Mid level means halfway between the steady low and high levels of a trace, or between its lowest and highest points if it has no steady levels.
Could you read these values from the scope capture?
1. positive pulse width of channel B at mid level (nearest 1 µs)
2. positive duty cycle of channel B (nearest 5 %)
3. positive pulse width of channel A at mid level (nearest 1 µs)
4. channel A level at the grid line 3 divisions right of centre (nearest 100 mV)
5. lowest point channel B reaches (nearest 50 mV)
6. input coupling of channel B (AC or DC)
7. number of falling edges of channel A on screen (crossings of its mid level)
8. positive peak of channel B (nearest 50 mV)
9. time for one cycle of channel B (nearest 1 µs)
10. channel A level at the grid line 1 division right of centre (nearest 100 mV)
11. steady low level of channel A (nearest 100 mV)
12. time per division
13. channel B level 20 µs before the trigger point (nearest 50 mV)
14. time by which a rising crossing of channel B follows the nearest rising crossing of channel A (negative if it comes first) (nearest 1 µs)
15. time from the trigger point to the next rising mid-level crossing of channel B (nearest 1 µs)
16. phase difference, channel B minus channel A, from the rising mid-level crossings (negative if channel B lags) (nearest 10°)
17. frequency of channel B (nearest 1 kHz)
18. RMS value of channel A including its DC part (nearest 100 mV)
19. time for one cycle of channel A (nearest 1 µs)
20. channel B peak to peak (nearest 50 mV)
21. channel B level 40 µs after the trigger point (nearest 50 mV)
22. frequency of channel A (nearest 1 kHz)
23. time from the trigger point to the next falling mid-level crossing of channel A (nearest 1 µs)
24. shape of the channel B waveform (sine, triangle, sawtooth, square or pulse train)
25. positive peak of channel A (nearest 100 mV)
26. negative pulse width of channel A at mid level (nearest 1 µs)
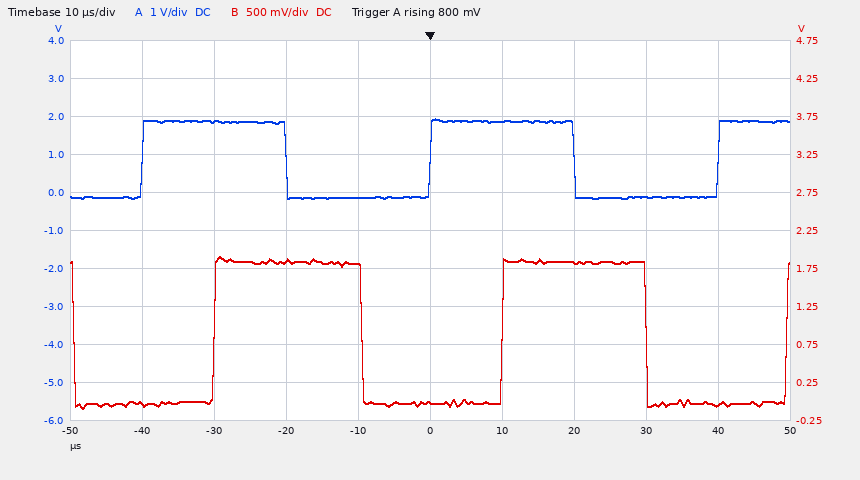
20 µs
50 %
20 µs
-100 mV
-100 mV
DC
2
1.90 V
40 µs
1.9 V
-100 mV
10 µs
1.85 V
+10 µs
10 µs
-90°
25 kHz
1.3 V
40 µs
2.00 V
-50 mV
25 kHz
20 µs
square
1.9 V
20 µs
